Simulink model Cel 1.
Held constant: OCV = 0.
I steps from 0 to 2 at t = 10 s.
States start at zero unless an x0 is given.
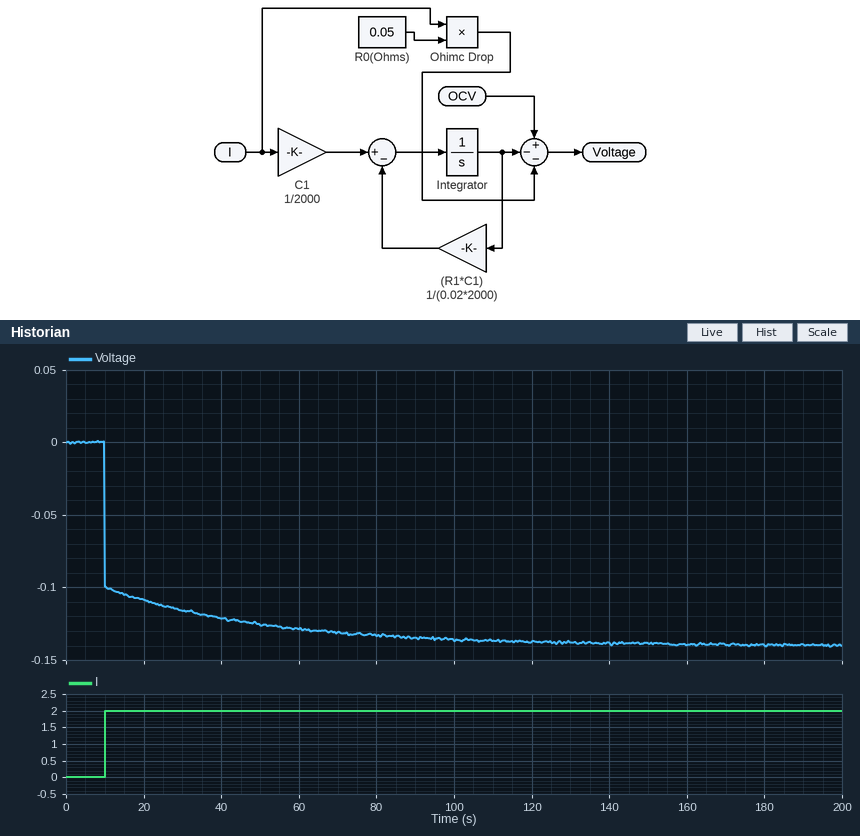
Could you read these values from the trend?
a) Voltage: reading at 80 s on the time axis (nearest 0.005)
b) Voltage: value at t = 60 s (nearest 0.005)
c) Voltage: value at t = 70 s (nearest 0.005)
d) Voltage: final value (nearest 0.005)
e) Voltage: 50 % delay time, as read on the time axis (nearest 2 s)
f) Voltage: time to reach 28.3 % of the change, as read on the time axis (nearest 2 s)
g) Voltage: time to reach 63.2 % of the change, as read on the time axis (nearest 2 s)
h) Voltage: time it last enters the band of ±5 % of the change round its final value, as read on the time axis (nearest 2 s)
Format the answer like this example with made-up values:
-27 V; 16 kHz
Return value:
-0.135; -0.130; -0.130; -0.140; 10 s; 10 s; 10 s; 80 s
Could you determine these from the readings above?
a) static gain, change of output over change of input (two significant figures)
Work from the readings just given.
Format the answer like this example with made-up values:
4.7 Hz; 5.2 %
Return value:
-0.070
